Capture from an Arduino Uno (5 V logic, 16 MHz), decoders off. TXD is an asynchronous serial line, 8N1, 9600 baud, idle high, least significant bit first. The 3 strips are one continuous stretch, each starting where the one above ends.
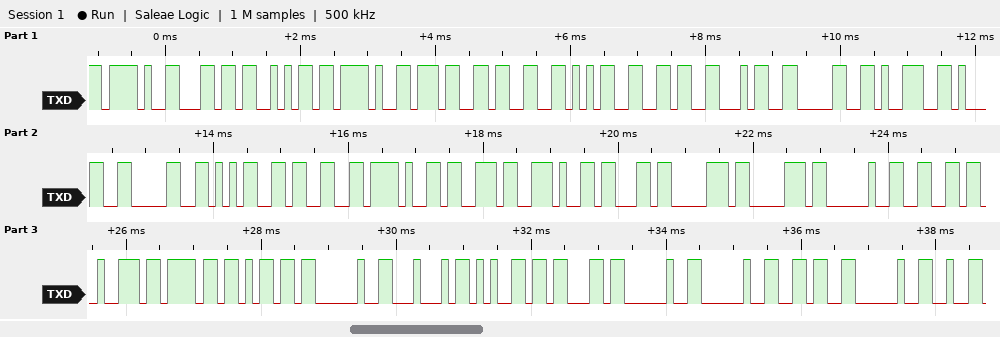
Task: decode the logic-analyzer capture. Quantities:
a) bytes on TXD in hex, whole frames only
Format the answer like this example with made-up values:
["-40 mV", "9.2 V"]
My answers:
["0x2F 0x6C 0x6A 0x2F 0x37 0x33 0x35 0x36 0x34 0x30 0x39 0x31 0x30 0x35 0x33 0x2F 0x73 0x2E 0x63 0x70 0x70 0x20 0x66 0x72 0x6F 0x6D 0x20 0x44 0x65 0x63 0x20 0x20 0x36 0x20"]
